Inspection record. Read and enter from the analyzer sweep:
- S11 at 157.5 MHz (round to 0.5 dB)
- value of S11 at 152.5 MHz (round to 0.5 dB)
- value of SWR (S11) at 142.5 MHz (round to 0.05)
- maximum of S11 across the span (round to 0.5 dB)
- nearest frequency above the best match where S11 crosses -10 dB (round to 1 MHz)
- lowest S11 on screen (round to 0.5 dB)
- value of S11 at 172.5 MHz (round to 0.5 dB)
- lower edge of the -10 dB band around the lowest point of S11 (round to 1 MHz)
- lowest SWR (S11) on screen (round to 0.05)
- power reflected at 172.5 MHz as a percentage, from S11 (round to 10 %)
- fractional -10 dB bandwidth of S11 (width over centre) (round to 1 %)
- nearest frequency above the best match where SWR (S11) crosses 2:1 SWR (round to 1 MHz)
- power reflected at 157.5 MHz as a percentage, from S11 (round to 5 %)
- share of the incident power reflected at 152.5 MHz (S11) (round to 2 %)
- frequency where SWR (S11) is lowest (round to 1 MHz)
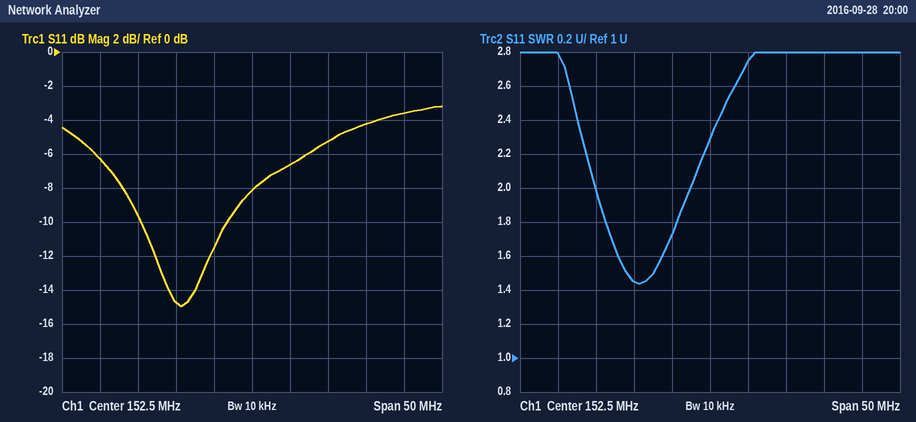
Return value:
-6.5 dB
-8.0 dB
1.45
-3.0 dB
149 MHz
-15.0 dB
-3.5 dB
138 MHz
1.45
40 %
8 %
150 MHz
20 %
16 %
143 MHz
